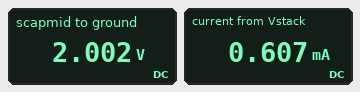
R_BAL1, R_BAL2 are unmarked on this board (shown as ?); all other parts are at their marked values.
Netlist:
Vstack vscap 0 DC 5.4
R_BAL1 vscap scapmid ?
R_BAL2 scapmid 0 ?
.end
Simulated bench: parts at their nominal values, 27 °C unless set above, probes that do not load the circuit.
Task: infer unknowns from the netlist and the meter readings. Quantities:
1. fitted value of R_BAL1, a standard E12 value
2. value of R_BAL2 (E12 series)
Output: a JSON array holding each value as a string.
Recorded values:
["5.6 kΩ", "3.3 kΩ"]
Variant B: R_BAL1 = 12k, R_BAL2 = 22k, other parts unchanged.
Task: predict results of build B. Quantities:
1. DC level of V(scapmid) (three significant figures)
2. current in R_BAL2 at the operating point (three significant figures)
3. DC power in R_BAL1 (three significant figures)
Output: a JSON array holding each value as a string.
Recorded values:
["3.49 V", "159 µA", "303 µW"]
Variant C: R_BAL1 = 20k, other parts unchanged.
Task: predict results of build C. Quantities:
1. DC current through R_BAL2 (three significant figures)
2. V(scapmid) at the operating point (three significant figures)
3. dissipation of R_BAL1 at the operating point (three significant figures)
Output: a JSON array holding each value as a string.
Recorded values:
["232 µA", "765 mV", "1.07 mW"]
